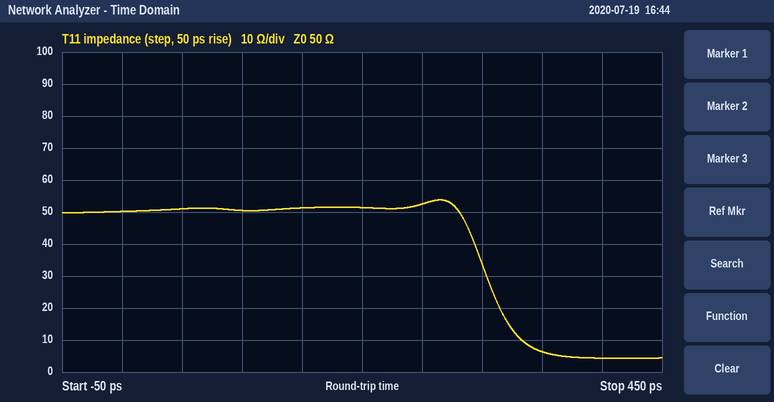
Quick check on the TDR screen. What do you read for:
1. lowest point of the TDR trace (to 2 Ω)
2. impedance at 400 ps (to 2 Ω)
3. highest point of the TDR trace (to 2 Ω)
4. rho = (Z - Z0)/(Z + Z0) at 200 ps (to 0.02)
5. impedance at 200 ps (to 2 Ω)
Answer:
4 Ω
4 Ω
54 Ω
+0.02
52 Ω
